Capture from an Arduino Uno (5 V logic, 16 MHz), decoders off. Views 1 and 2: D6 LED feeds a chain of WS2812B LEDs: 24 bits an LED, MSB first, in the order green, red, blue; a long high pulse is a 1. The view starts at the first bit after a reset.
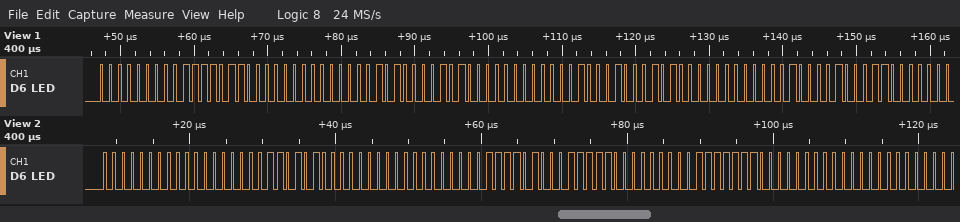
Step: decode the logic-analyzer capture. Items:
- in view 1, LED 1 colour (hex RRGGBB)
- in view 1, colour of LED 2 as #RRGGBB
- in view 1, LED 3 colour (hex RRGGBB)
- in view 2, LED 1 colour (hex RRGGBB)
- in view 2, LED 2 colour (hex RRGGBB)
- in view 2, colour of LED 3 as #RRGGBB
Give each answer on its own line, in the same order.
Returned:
#7B0000
#850200
#8A0800
#000035
#00003D
#001F7F
